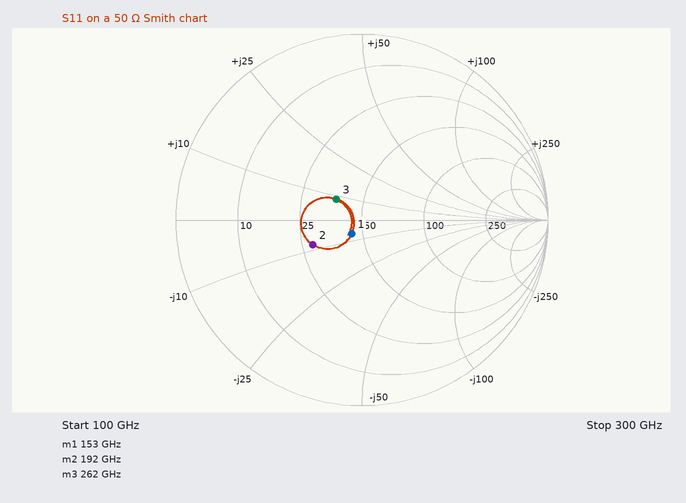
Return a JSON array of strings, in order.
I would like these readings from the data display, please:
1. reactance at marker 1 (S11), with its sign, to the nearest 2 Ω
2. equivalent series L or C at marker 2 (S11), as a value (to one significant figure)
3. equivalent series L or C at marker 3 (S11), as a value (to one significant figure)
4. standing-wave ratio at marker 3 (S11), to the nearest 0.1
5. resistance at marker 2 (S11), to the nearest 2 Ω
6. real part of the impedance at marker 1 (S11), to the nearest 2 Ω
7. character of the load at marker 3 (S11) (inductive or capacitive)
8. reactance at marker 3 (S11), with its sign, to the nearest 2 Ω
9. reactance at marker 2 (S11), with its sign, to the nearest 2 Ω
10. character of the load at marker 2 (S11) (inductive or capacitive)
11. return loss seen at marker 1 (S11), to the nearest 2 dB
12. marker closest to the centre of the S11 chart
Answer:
["-6 Ω", "100 fF", "5 pH", "1.4", "28 Ω", "44 Ω", "inductive", "+8 Ω", "-8 Ω", "capacitive", "20 dB", "marker 1"]
